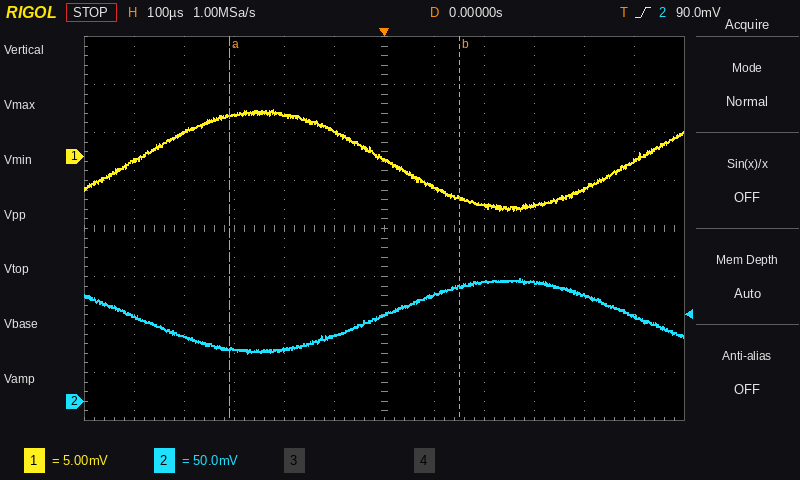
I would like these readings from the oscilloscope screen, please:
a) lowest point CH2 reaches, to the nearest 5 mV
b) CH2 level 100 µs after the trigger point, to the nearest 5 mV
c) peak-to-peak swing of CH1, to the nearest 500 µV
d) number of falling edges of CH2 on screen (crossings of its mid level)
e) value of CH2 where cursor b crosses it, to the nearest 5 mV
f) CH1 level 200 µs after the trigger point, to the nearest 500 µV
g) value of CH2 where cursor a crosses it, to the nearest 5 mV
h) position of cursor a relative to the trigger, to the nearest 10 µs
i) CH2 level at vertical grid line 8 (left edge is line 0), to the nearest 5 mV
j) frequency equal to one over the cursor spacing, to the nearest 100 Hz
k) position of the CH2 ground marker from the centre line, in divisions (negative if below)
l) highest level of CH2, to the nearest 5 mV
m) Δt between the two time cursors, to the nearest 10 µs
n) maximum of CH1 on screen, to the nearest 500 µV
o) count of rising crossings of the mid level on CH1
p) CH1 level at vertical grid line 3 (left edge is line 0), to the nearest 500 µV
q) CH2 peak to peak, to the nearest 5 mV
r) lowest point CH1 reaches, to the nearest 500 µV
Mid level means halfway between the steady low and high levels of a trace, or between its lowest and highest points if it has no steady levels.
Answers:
50 mV
110 mV
10.5 mV
2
120 mV
-5.0 mV
55 mV
-310 µs
125 mV
2.2 kHz
-3.6 div
130 mV
460 µs
5.0 mV
2
4.5 mV
80 mV
-5.5 mV
